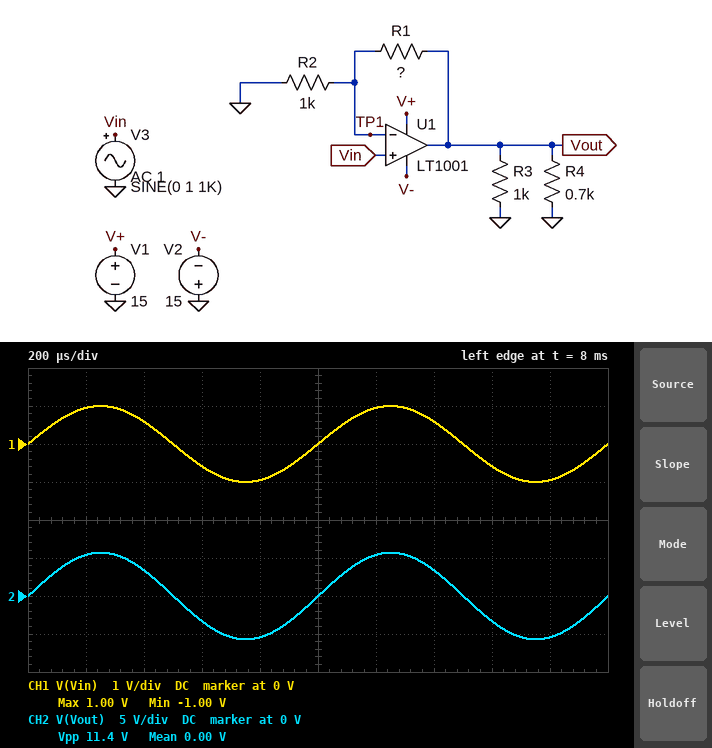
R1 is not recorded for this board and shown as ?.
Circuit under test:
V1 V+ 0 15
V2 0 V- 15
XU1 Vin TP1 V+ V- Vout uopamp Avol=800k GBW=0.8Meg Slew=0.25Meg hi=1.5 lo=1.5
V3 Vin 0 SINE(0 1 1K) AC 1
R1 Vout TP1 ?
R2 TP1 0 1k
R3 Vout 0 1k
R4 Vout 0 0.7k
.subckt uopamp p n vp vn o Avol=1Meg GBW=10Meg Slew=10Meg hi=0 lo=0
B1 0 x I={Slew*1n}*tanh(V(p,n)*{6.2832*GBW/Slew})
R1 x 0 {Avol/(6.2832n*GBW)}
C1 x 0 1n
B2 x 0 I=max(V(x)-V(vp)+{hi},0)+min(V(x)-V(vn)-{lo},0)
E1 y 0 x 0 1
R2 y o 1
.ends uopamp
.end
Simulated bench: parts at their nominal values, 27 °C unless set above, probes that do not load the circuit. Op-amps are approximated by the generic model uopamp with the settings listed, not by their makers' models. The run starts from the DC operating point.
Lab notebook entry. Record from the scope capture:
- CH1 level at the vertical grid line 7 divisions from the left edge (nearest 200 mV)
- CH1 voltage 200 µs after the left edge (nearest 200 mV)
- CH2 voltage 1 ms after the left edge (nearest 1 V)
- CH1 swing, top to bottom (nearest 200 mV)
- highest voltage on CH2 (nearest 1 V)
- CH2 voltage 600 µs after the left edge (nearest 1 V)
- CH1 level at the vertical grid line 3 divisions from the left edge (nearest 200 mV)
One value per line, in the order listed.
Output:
600 mV
1.0 V
0 V
2.0 V
6 V
-3 V
-600 mV
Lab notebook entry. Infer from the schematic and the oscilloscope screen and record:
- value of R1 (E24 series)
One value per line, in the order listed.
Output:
4.7 kΩ
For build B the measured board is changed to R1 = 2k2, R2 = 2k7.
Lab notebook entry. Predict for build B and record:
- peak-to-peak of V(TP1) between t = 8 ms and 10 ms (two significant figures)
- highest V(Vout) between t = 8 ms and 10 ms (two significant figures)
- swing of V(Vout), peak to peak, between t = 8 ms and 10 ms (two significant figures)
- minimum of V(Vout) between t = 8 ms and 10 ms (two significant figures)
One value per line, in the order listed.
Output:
2.0 V
1.8 V
3.6 V
-1.8 V
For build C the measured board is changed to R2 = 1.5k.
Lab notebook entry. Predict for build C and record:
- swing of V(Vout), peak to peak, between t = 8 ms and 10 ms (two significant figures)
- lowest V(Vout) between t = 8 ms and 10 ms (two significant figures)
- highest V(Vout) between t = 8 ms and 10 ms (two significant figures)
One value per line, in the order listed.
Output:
8.3 V
-4.1 V
4.1 V
